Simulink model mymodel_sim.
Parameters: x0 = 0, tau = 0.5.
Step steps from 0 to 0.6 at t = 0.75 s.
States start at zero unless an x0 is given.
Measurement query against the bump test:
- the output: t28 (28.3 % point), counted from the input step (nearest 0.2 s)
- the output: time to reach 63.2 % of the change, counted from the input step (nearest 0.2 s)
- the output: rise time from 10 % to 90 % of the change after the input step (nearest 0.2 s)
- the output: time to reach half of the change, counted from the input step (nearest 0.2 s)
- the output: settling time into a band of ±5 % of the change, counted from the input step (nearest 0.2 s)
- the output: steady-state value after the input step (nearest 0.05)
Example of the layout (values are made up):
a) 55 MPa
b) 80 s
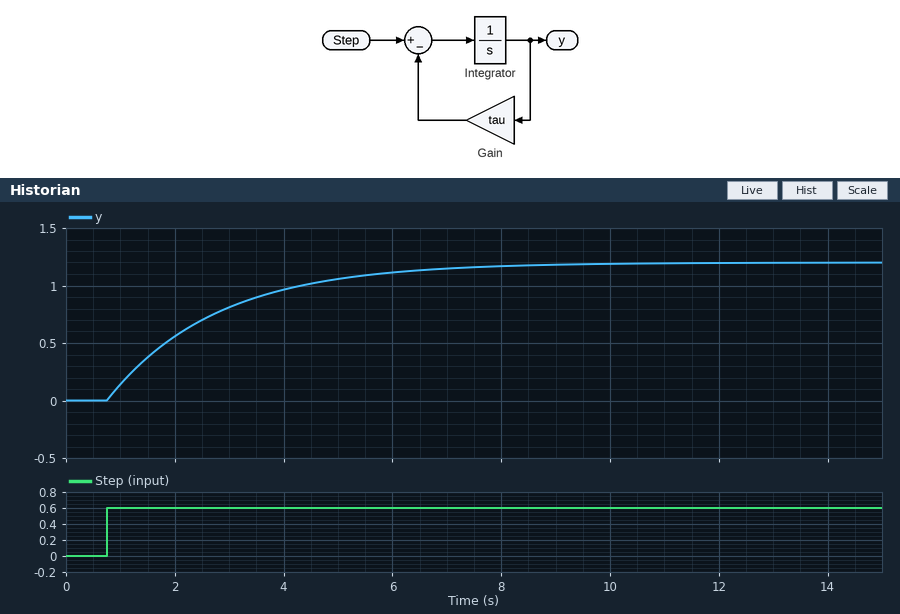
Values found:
a) 0.6 s
b) 2.0 s
c) 4.4 s
d) 1.4 s
e) 6.0 s
f) 1.20
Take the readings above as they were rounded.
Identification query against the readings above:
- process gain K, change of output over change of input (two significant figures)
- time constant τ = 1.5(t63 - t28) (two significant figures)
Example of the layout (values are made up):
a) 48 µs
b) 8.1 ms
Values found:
a) 2.0
b) 2.1 s
